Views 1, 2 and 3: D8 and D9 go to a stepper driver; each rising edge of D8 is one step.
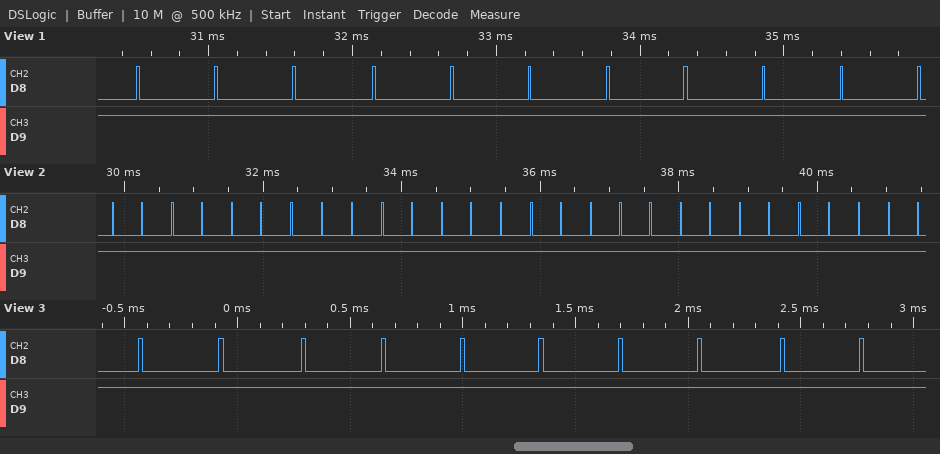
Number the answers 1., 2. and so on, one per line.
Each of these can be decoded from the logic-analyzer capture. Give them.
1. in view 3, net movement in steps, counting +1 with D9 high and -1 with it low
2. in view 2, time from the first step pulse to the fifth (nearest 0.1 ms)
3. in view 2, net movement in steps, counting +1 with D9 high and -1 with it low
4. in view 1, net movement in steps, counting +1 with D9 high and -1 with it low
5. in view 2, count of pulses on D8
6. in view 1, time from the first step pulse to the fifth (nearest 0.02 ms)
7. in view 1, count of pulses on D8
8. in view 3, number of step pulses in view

1. +10
2. 1.7 ms
3. +28
4. +11
5. 28
6. 2.18 ms
7. 11
8. 10
